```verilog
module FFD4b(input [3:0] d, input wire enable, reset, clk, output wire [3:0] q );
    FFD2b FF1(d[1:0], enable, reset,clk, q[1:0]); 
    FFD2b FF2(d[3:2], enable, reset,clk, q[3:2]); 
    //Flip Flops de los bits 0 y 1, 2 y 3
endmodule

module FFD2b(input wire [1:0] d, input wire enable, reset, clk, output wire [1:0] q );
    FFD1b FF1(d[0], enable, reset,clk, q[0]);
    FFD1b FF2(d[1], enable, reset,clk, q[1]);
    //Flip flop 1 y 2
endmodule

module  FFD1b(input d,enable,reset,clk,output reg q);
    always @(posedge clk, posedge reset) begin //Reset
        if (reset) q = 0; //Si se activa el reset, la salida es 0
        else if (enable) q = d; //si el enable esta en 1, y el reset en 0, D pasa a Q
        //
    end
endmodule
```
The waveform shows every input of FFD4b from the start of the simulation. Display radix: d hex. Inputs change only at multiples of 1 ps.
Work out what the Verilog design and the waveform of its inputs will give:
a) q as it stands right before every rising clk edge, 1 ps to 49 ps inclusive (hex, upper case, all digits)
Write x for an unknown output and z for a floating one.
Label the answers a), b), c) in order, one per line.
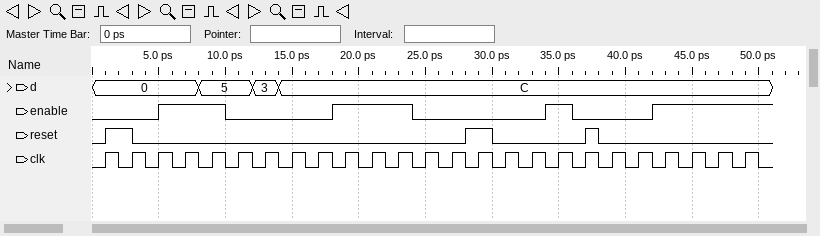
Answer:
a) x, 0, 0, 0, 0, 5, 5, 5, 5, 5, C, C, C, C, 0, 0, 0, 0, C, 0, 0, 0, C, C, C
